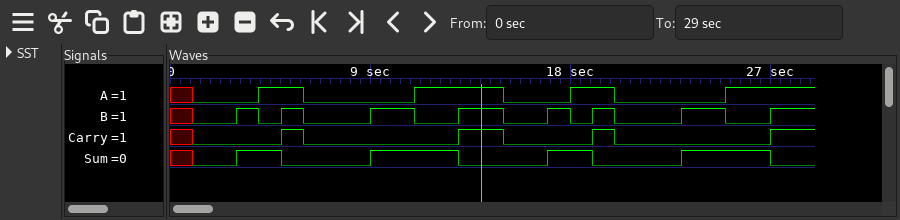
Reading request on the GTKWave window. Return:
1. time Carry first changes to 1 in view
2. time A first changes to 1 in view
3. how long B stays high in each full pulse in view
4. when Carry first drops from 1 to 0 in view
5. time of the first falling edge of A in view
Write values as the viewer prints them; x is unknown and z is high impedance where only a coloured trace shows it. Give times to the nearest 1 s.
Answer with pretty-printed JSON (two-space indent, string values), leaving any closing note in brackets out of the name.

{
  "time Carry first changes to 1 in view": "5 s",
  "time A first changes to 1 in view": "4 s",
  "how long B stays high in each full pulse in view": "1 s, 1 s, 2 s, 2 s, 1 s, 1 s, 2 s",
  "when Carry first drops from 1 to 0 in view": "6 s",
  "time of the first falling edge of A in view": "6 s"
}
